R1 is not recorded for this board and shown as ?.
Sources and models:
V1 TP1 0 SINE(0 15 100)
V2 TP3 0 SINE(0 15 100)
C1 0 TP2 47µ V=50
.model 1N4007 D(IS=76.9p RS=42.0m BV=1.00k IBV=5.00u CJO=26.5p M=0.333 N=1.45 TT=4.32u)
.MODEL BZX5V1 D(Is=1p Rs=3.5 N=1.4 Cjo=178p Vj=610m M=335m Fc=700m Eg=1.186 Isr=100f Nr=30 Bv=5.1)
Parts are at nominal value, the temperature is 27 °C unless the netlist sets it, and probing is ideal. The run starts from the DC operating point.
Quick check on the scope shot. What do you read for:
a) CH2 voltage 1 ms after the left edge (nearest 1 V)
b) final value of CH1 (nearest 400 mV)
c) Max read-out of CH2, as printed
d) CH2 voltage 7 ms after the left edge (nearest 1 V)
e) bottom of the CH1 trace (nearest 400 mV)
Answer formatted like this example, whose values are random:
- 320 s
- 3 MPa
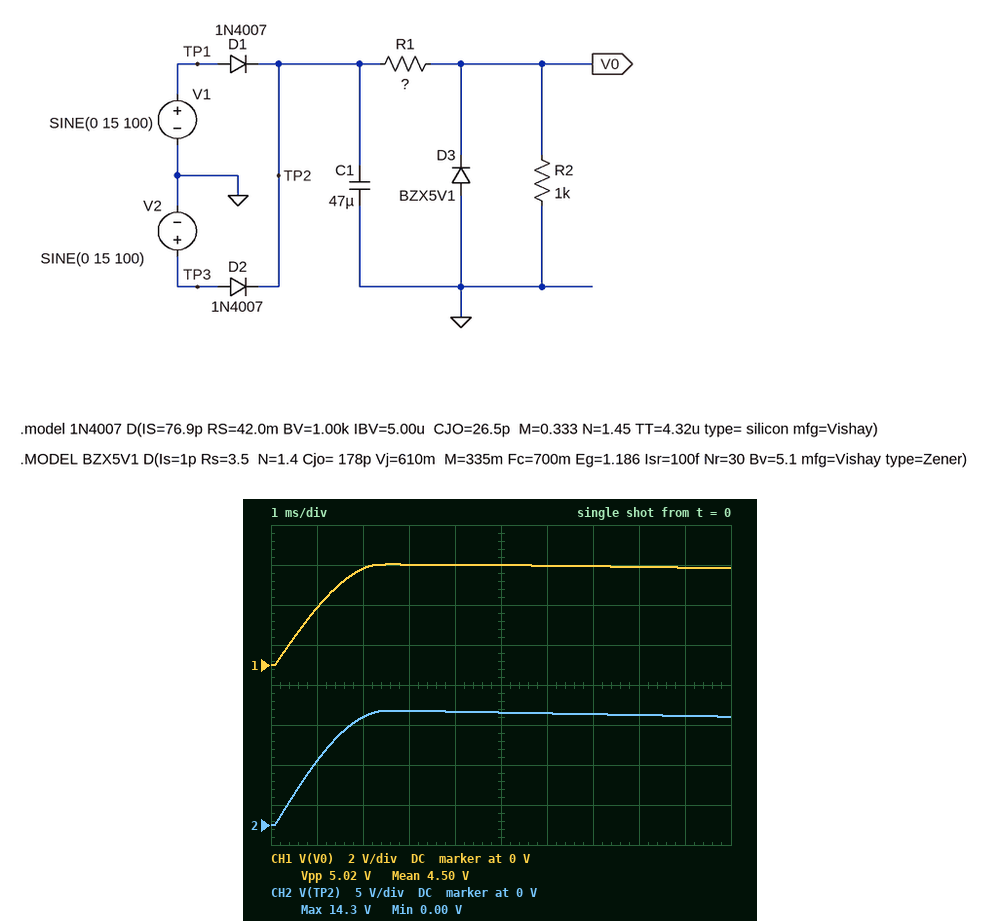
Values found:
- 8 V
- 4.8 V
- 14.3 V
- 14 V
- 0 V
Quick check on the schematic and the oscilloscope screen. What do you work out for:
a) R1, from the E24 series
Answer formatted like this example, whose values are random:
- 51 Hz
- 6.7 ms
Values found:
- 1.8 kΩ
